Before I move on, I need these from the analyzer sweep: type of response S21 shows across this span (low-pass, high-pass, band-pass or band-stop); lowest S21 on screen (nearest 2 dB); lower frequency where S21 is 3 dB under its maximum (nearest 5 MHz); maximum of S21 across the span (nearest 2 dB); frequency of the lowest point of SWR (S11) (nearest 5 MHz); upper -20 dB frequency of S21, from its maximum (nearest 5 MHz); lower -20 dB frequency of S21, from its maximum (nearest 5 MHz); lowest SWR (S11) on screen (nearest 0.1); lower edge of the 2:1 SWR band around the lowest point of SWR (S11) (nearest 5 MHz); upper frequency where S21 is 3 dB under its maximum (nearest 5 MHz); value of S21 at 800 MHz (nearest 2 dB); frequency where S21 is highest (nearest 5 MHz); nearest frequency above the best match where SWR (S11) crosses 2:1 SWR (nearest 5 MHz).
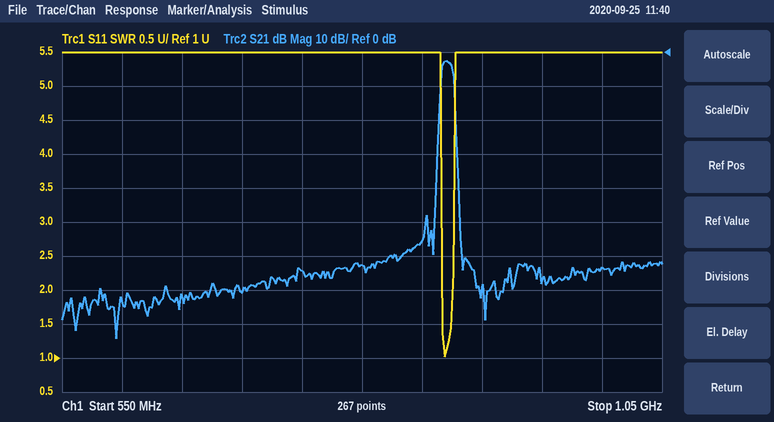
band-pass
-84 dB
865 MHz
-2 dB
870 MHz
880 MHz
865 MHz
1.0
865 MHz
875 MHz
-62 dB
870 MHz
875 MHz
